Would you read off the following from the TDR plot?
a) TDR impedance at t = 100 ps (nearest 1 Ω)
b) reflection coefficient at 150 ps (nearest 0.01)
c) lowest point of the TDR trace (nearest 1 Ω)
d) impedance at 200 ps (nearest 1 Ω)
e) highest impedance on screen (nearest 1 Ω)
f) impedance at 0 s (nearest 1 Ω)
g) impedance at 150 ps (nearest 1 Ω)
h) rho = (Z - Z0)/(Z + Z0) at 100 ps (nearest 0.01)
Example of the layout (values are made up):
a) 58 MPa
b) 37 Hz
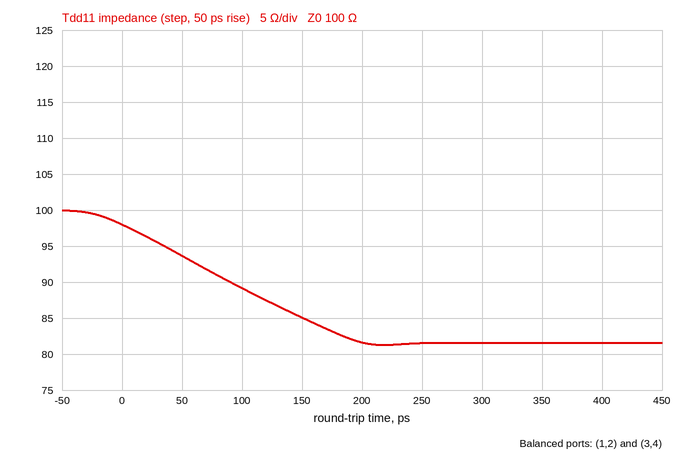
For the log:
a) 89 Ω
b) -0.08
c) 81 Ω
d) 82 Ω
e) 100 Ω
f) 98 Ω
g) 85 Ω
h) -0.06
